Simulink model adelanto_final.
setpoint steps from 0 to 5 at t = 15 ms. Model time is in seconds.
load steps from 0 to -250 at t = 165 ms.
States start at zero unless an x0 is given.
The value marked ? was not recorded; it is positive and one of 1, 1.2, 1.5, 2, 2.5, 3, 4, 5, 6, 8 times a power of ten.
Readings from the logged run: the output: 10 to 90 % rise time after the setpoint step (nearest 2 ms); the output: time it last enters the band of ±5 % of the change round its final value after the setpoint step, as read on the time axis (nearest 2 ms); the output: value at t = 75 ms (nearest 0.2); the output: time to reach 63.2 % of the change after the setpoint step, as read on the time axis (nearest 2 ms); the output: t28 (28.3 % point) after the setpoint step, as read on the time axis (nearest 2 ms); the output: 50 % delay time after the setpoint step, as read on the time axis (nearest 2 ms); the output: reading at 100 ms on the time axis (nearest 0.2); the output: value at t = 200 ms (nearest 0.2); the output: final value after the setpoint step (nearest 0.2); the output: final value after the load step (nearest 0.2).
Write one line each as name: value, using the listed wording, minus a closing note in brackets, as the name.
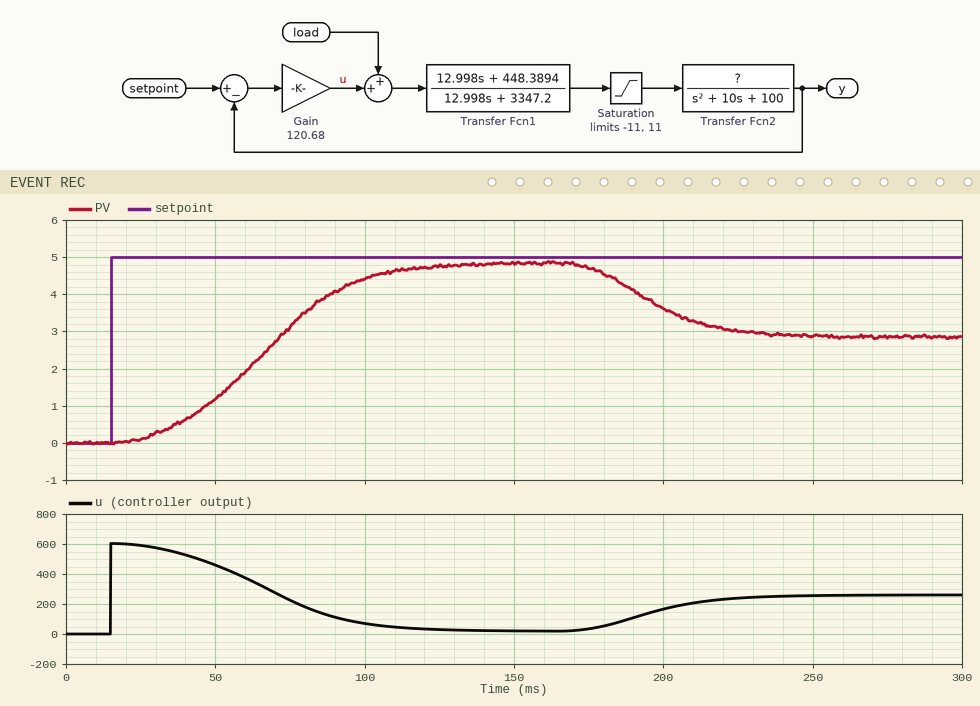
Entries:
the output: 10 to 90 % rise time after the setpoint step: 62 ms
the output: time it last enters the band of ±5 % of the change round its final value after the setpoint step, as read on the time axis: 110 ms
the output: value at t = 75 ms: 3.2
the output: time to reach 63.2 % of the change after the setpoint step, as read on the time axis: 74 ms
the output: t28 (28.3 % point) after the setpoint step, as read on the time axis: 52 ms
the output: 50 % delay time after the setpoint step, as read on the time axis: 66 ms
the output: reading at 100 ms on the time axis: 4.4
the output: value at t = 200 ms: 3.6
the output: final value after the setpoint step: 4.8
the output: final value after the load step: 2.8
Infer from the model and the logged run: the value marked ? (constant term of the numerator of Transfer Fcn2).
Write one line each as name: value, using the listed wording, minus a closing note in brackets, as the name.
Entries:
the value marked ?: 200
